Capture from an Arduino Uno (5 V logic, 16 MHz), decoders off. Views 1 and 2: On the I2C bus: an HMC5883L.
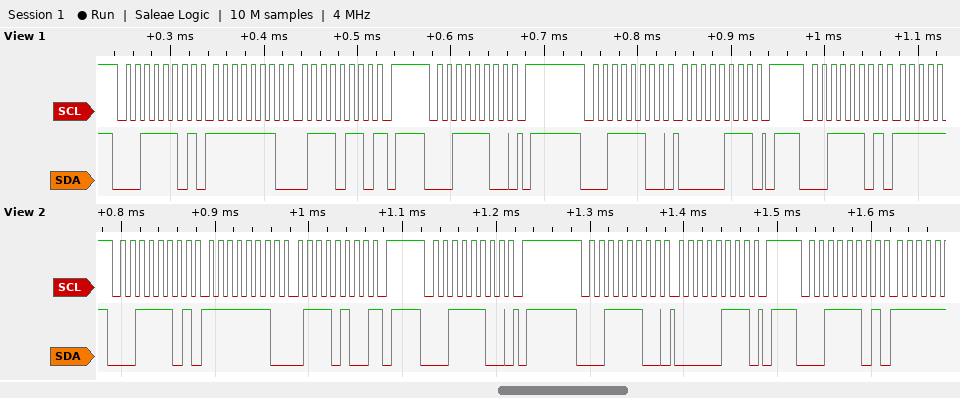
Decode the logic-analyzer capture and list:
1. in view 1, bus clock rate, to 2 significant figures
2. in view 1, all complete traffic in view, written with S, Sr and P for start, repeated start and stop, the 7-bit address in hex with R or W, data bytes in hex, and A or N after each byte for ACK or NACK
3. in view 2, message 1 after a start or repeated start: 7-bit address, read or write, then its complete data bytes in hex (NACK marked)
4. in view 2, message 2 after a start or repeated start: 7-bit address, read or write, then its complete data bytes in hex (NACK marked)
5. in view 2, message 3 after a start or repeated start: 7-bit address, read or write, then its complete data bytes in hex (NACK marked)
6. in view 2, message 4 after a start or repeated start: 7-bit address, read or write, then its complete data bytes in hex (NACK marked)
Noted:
100 kHz
S 1ER A FE A 76 N P S 1EW A P S 1EW A 07 A P S 1ER A
0x1E read: FE 74 NACK
0x1E write
0x1E write: 07
0x1E read
